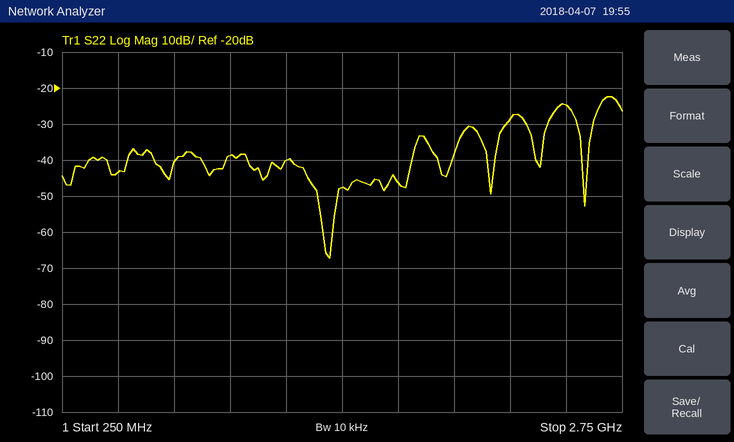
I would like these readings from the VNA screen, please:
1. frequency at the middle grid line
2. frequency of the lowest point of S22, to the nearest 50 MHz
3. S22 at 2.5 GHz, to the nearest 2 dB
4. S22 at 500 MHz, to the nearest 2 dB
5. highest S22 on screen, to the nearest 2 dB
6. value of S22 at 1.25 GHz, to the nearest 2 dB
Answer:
1.5 GHz
1.45 GHz
-24 dB
-44 dB
-22 dB
-40 dB
